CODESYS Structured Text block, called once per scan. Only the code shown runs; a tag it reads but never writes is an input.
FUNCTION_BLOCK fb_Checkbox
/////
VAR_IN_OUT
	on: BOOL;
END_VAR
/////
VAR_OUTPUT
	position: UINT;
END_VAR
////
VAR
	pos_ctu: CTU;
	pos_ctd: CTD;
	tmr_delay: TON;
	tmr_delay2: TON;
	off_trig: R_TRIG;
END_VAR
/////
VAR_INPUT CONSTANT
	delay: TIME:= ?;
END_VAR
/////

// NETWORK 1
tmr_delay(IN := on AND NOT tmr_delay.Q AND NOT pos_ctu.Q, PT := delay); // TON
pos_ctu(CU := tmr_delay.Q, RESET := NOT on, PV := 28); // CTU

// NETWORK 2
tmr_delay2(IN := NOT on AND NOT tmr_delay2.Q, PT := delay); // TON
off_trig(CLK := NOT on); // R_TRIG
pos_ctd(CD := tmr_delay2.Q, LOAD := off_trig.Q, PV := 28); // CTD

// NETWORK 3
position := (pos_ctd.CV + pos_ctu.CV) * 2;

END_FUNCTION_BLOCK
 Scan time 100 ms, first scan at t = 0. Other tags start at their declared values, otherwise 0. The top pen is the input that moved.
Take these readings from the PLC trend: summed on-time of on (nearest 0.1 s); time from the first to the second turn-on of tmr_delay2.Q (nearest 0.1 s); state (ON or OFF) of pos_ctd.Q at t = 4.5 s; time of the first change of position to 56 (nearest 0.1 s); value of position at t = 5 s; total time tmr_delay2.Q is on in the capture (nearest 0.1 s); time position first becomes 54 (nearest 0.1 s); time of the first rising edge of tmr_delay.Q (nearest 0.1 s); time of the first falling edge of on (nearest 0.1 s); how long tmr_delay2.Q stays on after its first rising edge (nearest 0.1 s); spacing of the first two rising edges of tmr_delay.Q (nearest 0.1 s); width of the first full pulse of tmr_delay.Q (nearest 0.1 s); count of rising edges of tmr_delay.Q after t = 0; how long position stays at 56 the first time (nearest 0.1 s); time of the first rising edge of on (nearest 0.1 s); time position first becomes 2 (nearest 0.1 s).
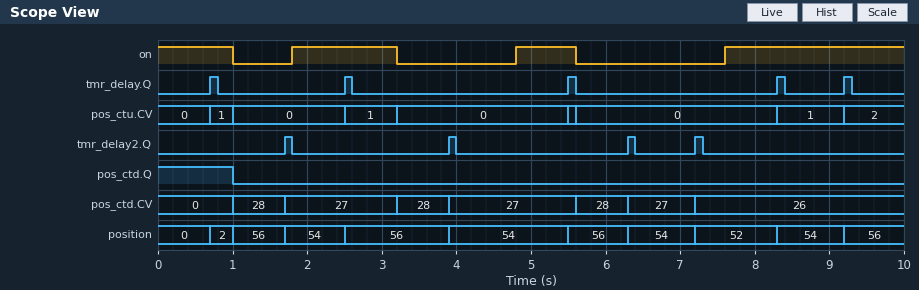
5.6 s
2.2 s
OFF
1.0 s
54
0.4 s
1.7 s
0.7 s
1.0 s
0.1 s
1.8 s
0.1 s
5
0.7 s
1.8 s
0.7 s
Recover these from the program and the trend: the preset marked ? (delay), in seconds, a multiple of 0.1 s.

0.7 s
